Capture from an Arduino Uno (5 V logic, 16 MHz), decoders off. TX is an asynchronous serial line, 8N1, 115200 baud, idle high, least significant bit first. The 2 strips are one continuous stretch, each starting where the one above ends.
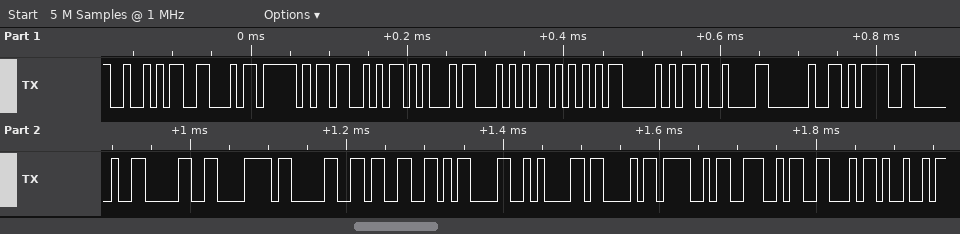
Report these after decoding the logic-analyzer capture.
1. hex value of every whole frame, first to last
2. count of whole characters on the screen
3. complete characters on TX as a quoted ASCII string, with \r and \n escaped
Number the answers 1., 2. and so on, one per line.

1. 0x52 0x46 0x5F 0x53 0x45 0x54 0x55 0x50 0x09 0x20 0x3D 0x20 0x30 0x78 0x30 0x33 0x0D 0x0A 0x43 0x4F 0x4E 0x46 0x49
2. 23
3. "RF_SETUP\t = 0x03\r\nCONFI"
